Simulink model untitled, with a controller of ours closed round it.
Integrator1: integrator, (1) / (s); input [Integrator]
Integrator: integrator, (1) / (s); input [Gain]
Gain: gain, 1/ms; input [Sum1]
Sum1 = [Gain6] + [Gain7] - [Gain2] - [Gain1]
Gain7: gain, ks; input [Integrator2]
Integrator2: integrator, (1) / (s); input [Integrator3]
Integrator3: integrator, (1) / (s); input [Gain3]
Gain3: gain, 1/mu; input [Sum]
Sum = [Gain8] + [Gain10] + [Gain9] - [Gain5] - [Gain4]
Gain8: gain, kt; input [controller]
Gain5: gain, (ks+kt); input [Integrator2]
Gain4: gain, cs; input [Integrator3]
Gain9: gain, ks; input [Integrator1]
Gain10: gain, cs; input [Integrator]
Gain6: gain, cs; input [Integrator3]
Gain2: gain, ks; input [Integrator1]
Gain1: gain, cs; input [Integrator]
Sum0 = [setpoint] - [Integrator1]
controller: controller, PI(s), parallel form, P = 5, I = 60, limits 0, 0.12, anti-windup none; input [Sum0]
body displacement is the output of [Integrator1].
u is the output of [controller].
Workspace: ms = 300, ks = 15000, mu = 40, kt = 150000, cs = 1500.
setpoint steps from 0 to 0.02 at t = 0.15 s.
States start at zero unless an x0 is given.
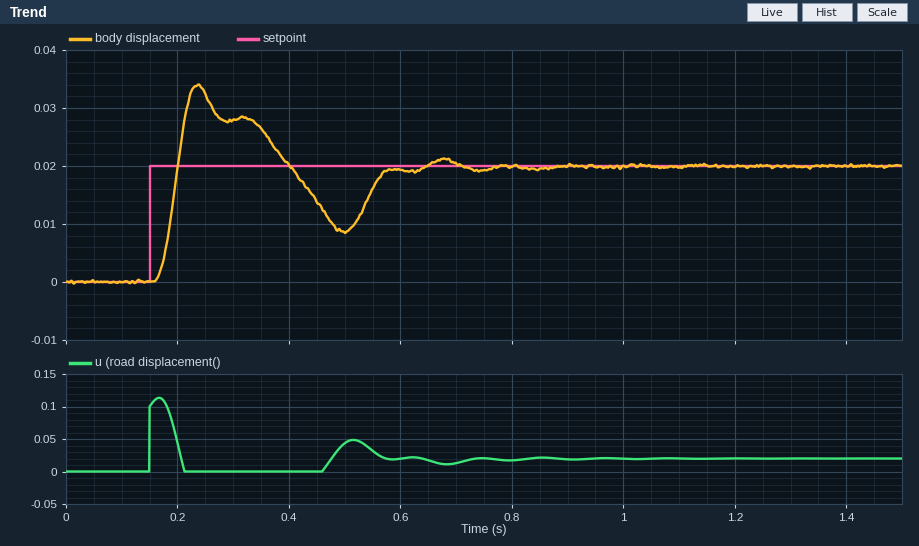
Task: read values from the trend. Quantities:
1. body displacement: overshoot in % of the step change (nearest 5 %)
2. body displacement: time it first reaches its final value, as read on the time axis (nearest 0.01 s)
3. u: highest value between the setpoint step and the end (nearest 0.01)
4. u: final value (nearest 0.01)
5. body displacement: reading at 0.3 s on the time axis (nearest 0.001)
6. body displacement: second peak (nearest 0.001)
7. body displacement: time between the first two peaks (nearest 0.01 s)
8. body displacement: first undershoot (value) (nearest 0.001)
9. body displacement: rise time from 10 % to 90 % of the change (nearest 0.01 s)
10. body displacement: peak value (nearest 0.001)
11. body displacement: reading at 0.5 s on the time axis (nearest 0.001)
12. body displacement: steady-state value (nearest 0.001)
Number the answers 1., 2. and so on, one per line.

1. 70 %
2. 0.20 s
3. 0.11
4. 0.02
5. 0.028
6. 0.021
7. 0.44 s
8. 0.009
9. 0.03 s
10. 0.034
11. 0.009
12. 0.020
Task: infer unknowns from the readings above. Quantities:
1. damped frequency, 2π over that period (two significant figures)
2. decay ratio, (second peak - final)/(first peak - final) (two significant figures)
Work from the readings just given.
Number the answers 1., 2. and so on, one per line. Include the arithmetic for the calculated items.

1. 2π / 0.44 = 14 rad/s
2. (0.021 - 0.02) / (0.034 - 0.02) = 0.071
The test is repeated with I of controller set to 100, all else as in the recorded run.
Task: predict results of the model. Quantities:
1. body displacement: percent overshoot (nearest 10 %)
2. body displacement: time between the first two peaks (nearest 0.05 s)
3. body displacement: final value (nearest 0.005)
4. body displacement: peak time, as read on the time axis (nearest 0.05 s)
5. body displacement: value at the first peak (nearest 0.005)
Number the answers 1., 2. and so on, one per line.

1. 100 %
2. 0.40 s
3. 0.020
4. 0.25 s
5. 0.040
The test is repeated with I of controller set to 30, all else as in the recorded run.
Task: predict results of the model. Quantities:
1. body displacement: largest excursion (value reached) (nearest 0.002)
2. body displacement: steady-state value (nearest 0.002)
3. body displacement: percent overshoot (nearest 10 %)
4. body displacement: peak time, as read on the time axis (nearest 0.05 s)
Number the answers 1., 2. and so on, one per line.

1. 0.030
2. 0.020
3. 50 %
4. 0.25 s
